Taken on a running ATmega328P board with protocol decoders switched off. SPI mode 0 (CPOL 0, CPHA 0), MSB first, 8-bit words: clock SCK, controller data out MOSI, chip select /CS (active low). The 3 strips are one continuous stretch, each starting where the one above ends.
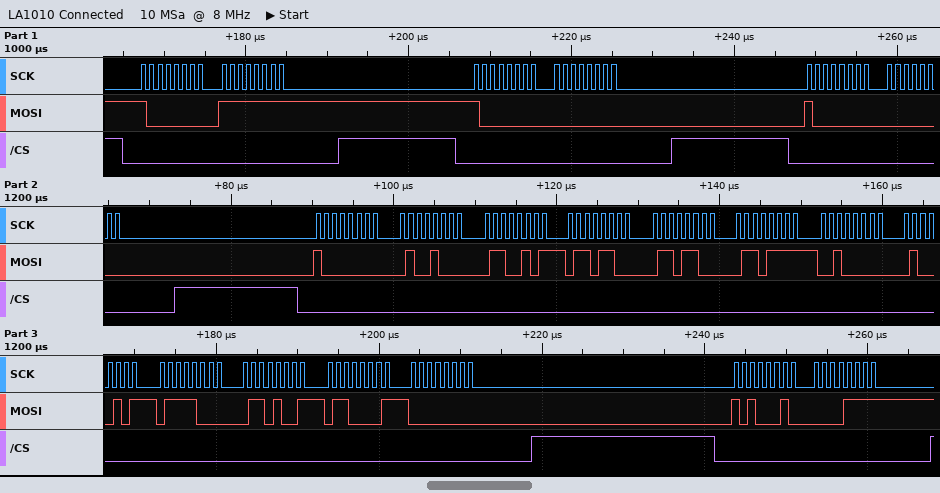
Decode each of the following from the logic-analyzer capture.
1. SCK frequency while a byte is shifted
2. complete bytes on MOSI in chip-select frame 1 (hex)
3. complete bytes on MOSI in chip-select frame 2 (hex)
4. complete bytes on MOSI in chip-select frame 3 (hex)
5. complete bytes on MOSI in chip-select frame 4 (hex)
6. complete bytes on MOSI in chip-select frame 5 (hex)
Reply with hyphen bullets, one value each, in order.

- 1 MHz
- 80 FF
- 80 00
- 80 00
- 80 48 65 6C 6C 6F 20 45 78 69 61 00
- A2 0F
